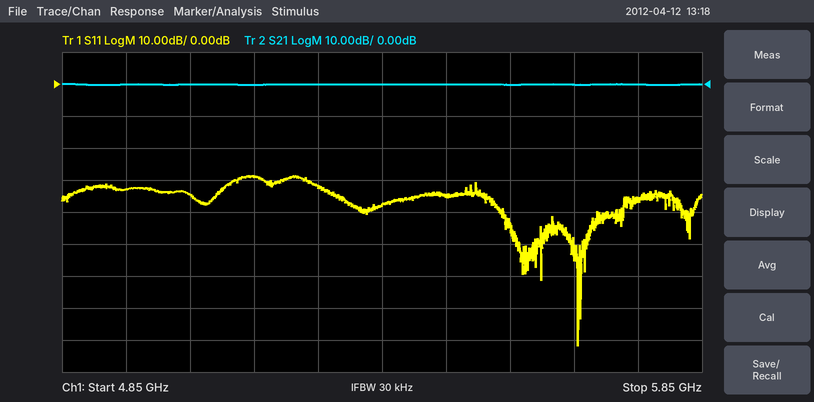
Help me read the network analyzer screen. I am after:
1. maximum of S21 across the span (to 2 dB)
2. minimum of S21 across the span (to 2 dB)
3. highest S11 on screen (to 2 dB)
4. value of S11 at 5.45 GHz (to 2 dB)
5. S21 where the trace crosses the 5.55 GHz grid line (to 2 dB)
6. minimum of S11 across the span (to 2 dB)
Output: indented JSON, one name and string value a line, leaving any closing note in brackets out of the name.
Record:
{
  "maximum of S21 across the span": "0 dB",
  "minimum of S21 across the span": "0 dB",
  "highest S11 on screen": "-28 dB",
  "value of S11 at 5.45 GHz": "-34 dB",
  "S21 where the trace crosses the 5.55 GHz grid line": "0 dB",
  "minimum of S11 across the span": "-82 dB"
}
